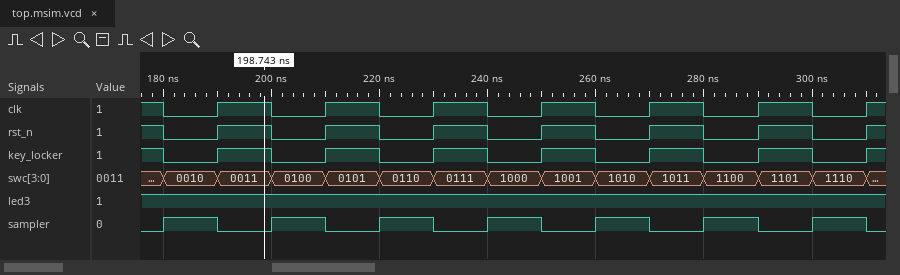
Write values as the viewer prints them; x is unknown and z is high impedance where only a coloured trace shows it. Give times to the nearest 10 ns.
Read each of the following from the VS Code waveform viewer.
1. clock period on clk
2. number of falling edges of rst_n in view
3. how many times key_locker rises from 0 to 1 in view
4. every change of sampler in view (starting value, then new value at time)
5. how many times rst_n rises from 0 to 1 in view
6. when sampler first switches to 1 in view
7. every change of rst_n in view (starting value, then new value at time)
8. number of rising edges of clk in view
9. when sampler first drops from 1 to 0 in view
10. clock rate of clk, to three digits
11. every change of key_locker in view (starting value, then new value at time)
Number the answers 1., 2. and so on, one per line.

1. 20 ns
2. 7
3. 7
4. 0, 1 at 180 ns, 0 at 190 ns, 1 at 200 ns, 0 at 210 ns, 1 at 220 ns, 0 at 230 ns, 1 at 240 ns, 0 at 250 ns, 1 at 260 ns, 0 at 270 ns, 1 at 280 ns, 0 at 290 ns, 1 at 300 ns, 0 at 310 ns
5. 7
6. 180 ns
7. 1, 0 at 180 ns, 1 at 190 ns, 0 at 200 ns, 1 at 210 ns, 0 at 220 ns, 1 at 230 ns, 0 at 240 ns, 1 at 250 ns, 0 at 260 ns, 1 at 270 ns, 0 at 280 ns, 1 at 290 ns, 0 at 300 ns, 1 at 310 ns
8. 7
9. 190 ns
10. 50.0 MHz
11. 1, 0 at 180 ns, 1 at 190 ns, 0 at 200 ns, 1 at 210 ns, 0 at 220 ns, 1 at 230 ns, 0 at 240 ns, 1 at 250 ns, 0 at 260 ns, 1 at 270 ns, 0 at 280 ns, 1 at 290 ns, 0 at 300 ns, 1 at 310 ns
